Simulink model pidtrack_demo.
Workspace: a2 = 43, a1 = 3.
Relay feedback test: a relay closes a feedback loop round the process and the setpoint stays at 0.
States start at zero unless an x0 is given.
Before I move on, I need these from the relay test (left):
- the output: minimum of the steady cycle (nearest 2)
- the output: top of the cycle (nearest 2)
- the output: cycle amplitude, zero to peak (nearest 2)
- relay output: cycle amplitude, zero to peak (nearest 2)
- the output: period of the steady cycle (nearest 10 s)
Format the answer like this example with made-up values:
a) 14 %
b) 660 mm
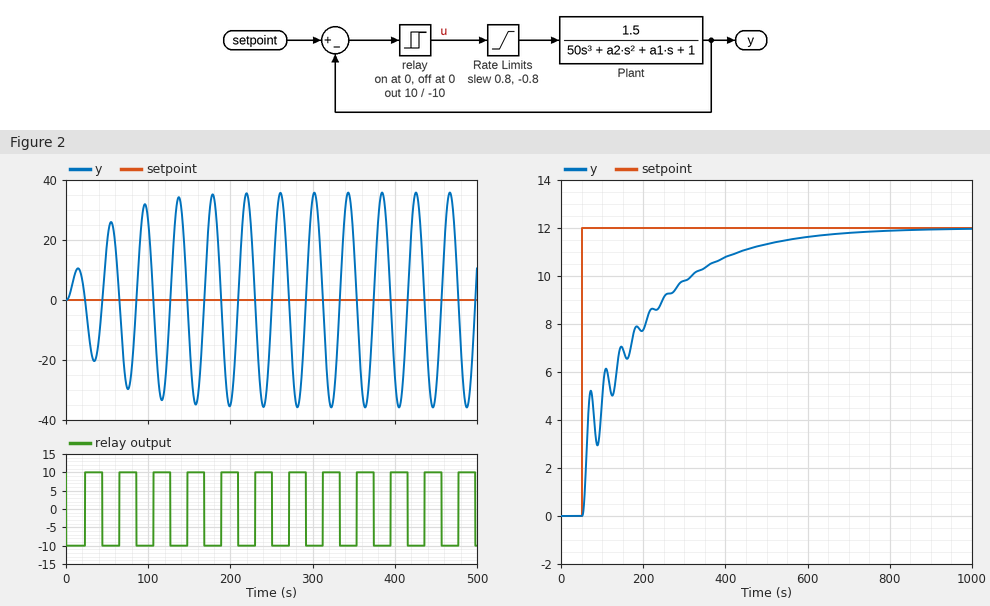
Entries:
a) -36
b) 36
c) 36
d) 10
e) 40 s
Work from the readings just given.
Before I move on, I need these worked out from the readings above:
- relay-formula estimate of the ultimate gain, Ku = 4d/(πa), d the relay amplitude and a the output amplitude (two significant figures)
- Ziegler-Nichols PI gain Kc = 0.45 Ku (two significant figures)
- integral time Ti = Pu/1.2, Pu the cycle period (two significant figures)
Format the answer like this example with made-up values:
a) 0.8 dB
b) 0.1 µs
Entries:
a) 0.35
b) 0.16
c) 33 s
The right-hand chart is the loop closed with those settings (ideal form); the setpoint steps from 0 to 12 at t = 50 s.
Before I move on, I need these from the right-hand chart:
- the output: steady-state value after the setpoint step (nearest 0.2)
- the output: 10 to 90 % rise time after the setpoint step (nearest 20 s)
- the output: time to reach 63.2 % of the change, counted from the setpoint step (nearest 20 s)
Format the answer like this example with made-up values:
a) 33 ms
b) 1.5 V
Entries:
a) 12.0
b) 340 s
c) 120 s
